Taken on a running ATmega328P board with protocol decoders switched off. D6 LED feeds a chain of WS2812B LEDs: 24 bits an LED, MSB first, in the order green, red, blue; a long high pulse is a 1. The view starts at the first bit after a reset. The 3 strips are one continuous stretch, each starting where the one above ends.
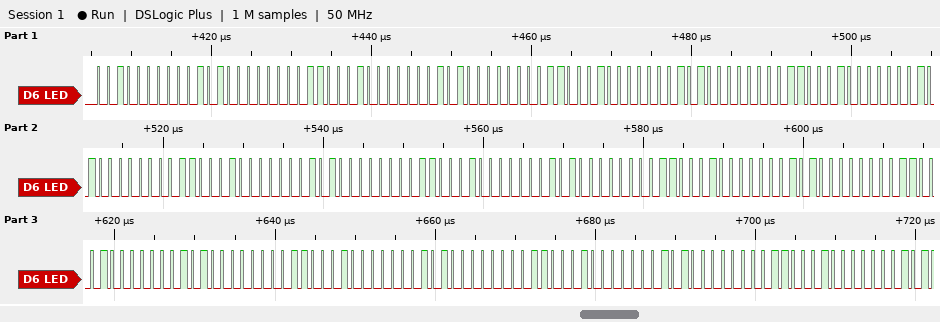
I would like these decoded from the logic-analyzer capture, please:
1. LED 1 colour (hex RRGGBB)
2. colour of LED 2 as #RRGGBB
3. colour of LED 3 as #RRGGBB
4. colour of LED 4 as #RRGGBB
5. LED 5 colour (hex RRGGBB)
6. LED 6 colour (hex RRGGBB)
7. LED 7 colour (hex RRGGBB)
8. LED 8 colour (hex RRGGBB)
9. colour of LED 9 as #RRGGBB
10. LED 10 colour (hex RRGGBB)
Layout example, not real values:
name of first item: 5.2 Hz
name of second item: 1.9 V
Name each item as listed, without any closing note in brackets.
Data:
LED 1 colour: #282006
colour of LED 2 as #RRGGBB: #282006
colour of LED 3 as #RRGGBB: #282006
colour of LED 4 as #RRGGBB: #282006
LED 5 colour: #282006
LED 6 colour: #282006
LED 7 colour: #282006
LED 8 colour: #282006
colour of LED 9 as #RRGGBB: #282006
LED 10 colour: #282006
